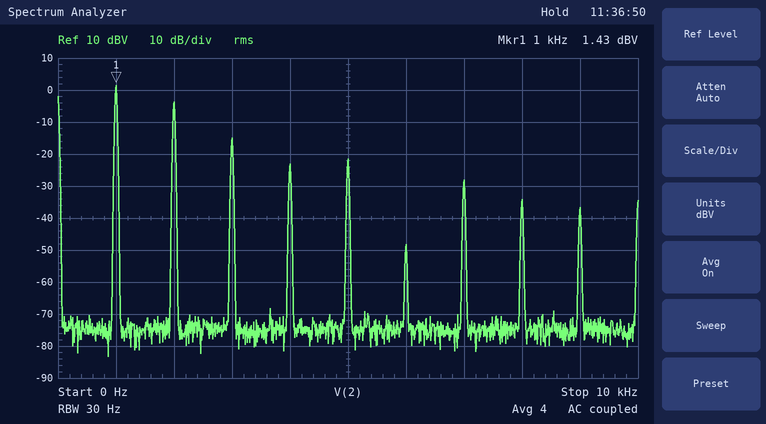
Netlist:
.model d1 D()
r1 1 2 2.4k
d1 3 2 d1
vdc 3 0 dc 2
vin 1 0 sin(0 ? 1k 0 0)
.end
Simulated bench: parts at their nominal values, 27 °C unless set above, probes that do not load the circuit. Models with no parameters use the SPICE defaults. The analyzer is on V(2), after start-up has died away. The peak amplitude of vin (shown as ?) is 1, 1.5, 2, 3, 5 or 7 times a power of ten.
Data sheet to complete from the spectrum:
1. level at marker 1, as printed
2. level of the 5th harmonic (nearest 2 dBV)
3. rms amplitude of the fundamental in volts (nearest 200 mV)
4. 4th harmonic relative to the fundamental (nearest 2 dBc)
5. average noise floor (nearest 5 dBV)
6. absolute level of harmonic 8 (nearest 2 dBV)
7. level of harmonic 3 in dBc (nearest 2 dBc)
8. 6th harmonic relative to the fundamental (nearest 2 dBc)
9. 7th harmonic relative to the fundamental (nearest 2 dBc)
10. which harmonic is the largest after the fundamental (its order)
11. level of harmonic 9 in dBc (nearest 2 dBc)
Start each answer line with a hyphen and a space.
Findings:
- 1.43 dBV
- -22 dBV
- 1.2 V
- -24 dBc
- -75 dBV
- -34 dBV
- -16 dBc
- -50 dBc
- -30 dBc
- 2
- -38 dBc
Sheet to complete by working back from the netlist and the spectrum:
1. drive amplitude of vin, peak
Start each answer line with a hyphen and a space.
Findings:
- 5 V
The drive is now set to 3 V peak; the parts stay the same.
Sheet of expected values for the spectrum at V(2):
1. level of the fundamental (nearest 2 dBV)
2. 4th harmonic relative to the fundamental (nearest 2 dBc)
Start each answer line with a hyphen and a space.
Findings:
- -6 dBV
- -30 dBc
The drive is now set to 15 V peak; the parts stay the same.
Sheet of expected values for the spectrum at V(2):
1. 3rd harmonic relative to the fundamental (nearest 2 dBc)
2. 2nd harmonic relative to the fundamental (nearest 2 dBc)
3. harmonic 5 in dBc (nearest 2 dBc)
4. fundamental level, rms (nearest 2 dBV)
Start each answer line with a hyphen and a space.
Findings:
- -28 dBc
- -6 dBc
- -32 dBc
- 14 dBV
